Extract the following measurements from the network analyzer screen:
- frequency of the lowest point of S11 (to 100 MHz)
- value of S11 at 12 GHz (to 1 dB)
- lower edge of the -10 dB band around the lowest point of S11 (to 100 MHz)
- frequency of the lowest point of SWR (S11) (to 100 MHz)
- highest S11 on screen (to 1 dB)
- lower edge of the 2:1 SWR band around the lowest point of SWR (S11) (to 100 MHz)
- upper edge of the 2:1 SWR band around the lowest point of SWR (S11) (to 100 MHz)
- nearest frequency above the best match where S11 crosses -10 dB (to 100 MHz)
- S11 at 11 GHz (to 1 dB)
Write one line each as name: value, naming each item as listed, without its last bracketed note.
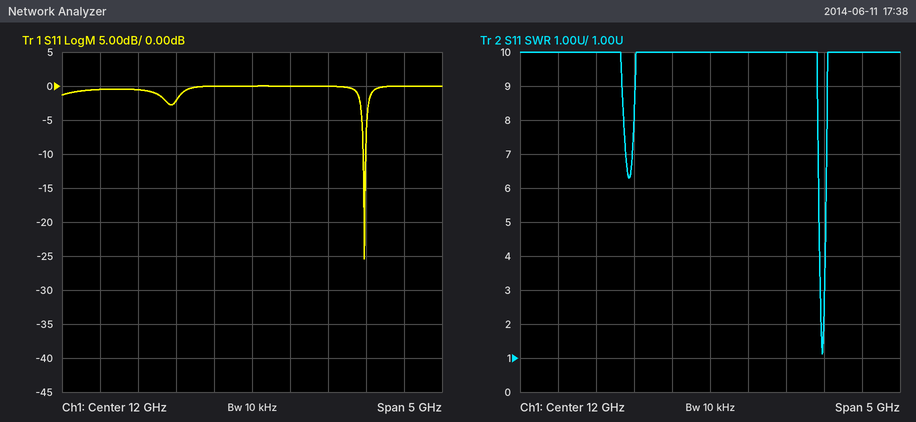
frequency of the lowest point of S11: 13.5 GHz
value of S11 at 12 GHz: 0 dB
lower edge of the -10 dB band around the lowest point of S11: 13.5 GHz
frequency of the lowest point of SWR (S11): 13.5 GHz
highest S11 on screen: 0 dB
lower edge of the 2:1 SWR band around the lowest point of SWR (S11): 13.5 GHz
upper edge of the 2:1 SWR band around the lowest point of SWR (S11): 13.5 GHz
nearest frequency above the best match where S11 crosses -10 dB: 13.5 GHz
S11 at 11 GHz: -2 dB
